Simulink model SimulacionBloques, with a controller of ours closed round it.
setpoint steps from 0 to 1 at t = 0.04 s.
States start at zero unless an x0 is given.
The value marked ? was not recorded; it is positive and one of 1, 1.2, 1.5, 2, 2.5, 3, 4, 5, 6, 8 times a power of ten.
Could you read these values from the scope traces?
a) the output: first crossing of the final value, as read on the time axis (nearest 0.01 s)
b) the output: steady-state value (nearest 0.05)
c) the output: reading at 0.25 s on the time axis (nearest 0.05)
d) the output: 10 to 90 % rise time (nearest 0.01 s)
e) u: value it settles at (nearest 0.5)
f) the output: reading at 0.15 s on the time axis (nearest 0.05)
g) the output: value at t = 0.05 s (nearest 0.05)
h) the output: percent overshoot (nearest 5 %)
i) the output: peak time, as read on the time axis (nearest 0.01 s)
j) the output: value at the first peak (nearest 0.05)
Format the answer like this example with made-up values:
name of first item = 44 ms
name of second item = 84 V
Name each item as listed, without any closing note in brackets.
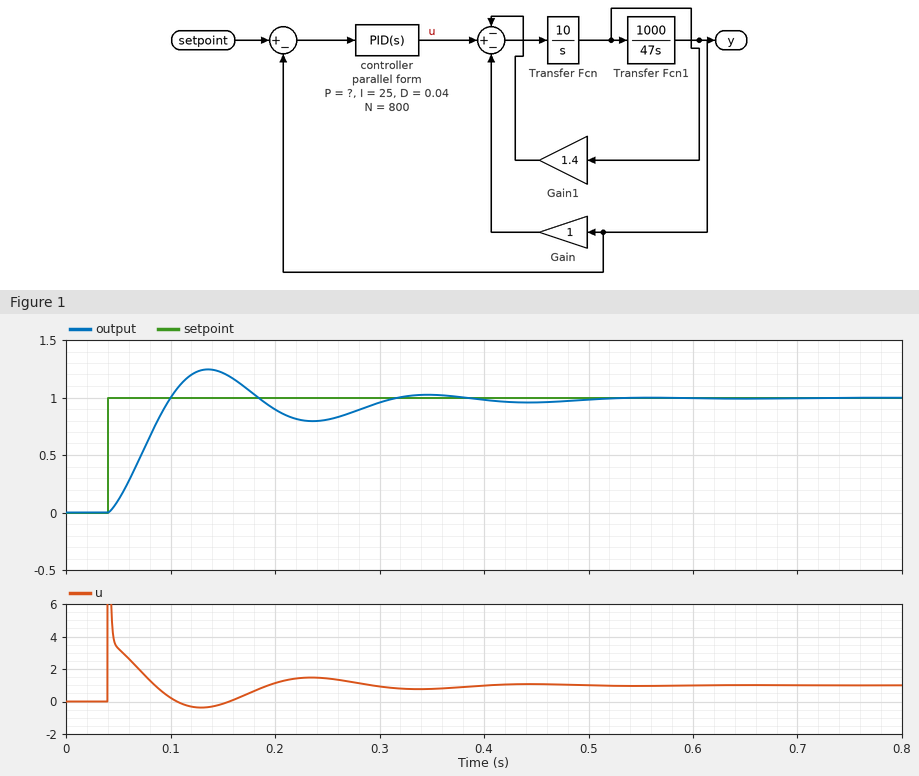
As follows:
the output: first crossing of the final value, as read on the time axis = 0.10 s
the output: steady-state value = 1.00
the output: reading at 0.25 s on the time axis = 0.80
the output: 10 to 90 % rise time = 0.04 s
u: value it settles at = 1.0
the output: reading at 0.15 s on the time axis = 1.20
the output: value at t = 0.05 s = 0.10
the output: percent overshoot = 25 %
the output: peak time, as read on the time axis = 0.14 s
the output: value at the first peak = 1.25
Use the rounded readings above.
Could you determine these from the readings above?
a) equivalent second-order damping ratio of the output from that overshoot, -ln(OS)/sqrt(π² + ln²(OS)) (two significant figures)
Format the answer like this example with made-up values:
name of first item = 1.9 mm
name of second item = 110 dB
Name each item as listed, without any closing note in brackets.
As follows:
equivalent second-order damping ratio of the output from that overshoot, -ln(OS)/sqrt(π² + ln²(OS)) = 0.40
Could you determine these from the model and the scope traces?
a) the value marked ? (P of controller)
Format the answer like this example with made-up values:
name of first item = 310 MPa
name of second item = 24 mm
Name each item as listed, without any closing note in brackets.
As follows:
the value marked ? = 4
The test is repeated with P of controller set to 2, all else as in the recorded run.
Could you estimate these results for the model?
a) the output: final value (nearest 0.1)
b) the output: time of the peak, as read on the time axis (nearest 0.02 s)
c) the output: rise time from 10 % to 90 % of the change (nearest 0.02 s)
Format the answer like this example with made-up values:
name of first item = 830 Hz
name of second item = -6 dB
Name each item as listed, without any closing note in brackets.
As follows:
the output: final value = 1.0
the output: time of the peak, as read on the time axis = 0.18 s
the output: rise time from 10 % to 90 % of the change = 0.06 s
